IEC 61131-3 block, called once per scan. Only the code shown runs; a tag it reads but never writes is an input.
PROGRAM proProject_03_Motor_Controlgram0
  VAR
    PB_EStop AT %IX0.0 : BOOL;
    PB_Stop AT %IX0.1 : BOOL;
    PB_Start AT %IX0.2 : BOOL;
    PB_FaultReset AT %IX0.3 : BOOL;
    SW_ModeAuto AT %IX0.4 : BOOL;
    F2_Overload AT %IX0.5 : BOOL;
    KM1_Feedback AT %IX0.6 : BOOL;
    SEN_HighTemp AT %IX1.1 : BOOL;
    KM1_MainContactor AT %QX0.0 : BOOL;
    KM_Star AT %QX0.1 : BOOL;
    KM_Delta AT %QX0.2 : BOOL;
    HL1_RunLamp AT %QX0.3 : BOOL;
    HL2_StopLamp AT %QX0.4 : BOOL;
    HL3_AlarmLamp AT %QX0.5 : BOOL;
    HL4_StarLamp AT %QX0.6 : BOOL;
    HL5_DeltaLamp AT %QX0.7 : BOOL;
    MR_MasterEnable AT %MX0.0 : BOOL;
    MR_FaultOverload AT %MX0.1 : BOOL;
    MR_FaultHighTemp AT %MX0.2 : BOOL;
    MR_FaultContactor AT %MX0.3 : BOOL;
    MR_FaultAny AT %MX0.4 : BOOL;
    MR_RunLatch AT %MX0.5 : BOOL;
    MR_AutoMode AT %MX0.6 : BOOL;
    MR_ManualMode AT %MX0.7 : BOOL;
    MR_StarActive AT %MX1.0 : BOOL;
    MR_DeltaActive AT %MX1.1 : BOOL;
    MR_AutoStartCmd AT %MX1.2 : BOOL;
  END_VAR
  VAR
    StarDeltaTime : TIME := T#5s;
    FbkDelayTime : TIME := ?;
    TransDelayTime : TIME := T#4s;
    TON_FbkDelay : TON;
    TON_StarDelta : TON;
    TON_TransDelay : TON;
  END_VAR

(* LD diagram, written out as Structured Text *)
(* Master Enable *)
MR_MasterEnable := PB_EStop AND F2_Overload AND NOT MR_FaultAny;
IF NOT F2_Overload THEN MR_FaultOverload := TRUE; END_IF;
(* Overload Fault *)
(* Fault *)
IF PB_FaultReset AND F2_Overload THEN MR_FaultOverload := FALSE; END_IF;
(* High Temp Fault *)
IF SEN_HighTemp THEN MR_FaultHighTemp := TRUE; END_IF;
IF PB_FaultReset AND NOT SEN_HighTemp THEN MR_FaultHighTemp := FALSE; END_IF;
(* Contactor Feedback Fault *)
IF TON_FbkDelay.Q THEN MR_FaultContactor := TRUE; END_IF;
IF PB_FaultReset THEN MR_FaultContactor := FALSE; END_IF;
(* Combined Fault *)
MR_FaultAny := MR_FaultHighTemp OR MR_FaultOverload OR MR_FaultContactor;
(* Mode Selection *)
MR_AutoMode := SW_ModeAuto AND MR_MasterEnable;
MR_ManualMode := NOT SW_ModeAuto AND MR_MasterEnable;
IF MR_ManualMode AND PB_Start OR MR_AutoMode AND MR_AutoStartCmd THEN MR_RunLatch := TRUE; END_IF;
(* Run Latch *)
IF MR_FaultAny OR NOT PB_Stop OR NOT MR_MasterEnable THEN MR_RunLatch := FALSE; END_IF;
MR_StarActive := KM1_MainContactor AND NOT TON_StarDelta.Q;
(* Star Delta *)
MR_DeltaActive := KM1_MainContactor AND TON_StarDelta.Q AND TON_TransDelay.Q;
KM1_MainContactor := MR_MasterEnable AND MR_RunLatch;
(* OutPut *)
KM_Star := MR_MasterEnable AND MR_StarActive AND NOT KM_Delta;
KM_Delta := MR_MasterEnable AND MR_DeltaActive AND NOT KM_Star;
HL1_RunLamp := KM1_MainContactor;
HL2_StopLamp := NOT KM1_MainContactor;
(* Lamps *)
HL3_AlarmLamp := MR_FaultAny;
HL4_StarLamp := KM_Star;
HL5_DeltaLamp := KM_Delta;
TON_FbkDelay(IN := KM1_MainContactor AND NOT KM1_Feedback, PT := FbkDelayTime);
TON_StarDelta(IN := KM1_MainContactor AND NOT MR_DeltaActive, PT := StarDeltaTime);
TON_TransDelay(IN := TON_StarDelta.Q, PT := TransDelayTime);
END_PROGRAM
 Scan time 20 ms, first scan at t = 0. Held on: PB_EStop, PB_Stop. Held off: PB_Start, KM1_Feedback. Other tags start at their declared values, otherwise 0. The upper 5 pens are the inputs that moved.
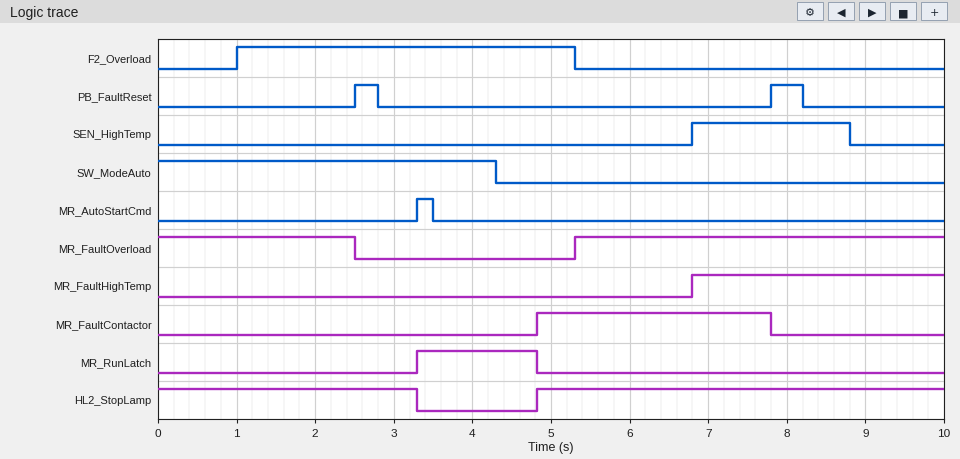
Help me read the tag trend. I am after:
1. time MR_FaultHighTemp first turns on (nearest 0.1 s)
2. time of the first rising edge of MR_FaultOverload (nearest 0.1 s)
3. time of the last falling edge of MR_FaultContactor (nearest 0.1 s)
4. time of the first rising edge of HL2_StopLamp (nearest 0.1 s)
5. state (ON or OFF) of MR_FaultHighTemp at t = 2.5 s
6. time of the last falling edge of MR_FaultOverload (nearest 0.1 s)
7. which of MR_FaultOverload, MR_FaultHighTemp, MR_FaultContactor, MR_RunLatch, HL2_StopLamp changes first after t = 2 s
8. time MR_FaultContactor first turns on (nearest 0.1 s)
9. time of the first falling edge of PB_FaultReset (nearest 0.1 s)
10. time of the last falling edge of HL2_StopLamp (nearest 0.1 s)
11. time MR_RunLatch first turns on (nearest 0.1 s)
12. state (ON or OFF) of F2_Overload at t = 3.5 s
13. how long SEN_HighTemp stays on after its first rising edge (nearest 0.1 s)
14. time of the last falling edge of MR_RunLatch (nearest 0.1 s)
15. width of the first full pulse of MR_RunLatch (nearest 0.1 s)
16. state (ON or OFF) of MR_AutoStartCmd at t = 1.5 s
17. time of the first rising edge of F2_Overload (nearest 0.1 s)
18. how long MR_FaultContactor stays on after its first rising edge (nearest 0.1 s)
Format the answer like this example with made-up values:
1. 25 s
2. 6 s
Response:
1. 6.8 s
2. 5.3 s
3. 7.8 s
4. 4.8 s
5. OFF
6. 2.5 s
7. MR_FaultOverload
8. 4.8 s
9. 2.8 s
10. 3.3 s
11. 3.3 s
12. ON
13. 2.0 s
14. 4.8 s
15. 1.5 s
16. OFF
17. 1.0 s
18. 3.0 s
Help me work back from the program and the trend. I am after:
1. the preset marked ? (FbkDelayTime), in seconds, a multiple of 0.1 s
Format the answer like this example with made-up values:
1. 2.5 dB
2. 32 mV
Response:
1. 1.5 s
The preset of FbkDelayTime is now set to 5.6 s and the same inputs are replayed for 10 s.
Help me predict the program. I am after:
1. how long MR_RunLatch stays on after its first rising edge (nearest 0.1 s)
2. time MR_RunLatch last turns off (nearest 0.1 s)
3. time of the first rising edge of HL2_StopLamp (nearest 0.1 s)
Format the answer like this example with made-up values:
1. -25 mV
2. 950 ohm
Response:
1. 2.0 s
2. 5.3 s
3. 5.3 s
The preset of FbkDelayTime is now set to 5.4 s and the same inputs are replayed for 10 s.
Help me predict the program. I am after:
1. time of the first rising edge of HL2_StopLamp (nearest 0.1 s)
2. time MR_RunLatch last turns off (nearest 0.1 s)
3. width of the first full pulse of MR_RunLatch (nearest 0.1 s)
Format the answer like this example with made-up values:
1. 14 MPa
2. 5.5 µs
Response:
1. 5.3 s
2. 5.3 s
3. 2.0 s
